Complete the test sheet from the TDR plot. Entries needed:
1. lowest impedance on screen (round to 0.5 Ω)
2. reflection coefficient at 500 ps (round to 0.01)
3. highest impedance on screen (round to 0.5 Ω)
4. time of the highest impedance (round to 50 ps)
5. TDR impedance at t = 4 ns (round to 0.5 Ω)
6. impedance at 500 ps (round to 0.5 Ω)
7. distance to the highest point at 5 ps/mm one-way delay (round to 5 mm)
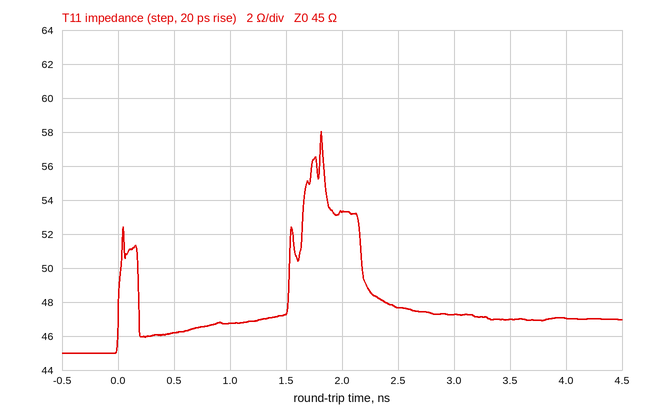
45.0 Ω
+0.01
58.0 Ω
1.80 ns
47.0 Ω
46.0 Ω
180 mm
